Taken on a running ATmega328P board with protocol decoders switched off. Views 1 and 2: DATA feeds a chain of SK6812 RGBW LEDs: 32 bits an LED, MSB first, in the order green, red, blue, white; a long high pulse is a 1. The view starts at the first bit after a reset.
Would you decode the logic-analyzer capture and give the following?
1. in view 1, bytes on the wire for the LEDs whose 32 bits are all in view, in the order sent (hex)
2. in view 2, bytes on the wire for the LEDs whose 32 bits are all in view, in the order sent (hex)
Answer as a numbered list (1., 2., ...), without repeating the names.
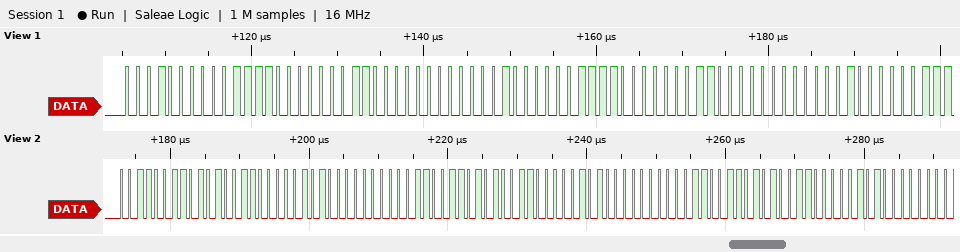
1. 10 3C 06 00 10 3C 06 00
2. 33 53 05 00 33 53 05 00 33 53 05 00
